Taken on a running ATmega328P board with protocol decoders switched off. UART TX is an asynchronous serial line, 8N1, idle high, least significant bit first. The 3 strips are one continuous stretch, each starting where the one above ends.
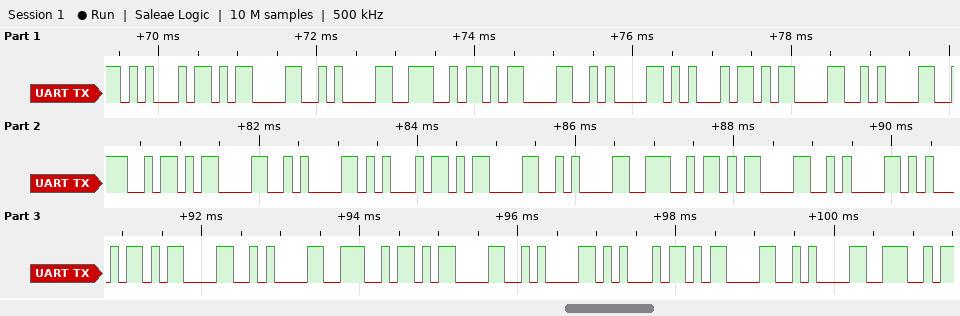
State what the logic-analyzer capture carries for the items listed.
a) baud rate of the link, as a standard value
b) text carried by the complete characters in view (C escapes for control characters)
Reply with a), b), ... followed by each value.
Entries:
a) 9600 baud
b) "E\r\nN\r\nE\r\nN\r\nE\r\nN\r\nE\r\nN\r\nE\r\nN"
